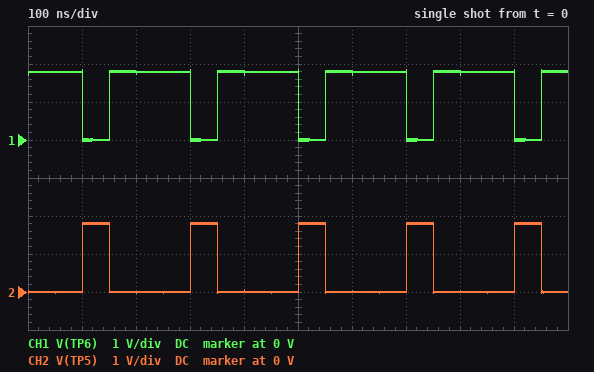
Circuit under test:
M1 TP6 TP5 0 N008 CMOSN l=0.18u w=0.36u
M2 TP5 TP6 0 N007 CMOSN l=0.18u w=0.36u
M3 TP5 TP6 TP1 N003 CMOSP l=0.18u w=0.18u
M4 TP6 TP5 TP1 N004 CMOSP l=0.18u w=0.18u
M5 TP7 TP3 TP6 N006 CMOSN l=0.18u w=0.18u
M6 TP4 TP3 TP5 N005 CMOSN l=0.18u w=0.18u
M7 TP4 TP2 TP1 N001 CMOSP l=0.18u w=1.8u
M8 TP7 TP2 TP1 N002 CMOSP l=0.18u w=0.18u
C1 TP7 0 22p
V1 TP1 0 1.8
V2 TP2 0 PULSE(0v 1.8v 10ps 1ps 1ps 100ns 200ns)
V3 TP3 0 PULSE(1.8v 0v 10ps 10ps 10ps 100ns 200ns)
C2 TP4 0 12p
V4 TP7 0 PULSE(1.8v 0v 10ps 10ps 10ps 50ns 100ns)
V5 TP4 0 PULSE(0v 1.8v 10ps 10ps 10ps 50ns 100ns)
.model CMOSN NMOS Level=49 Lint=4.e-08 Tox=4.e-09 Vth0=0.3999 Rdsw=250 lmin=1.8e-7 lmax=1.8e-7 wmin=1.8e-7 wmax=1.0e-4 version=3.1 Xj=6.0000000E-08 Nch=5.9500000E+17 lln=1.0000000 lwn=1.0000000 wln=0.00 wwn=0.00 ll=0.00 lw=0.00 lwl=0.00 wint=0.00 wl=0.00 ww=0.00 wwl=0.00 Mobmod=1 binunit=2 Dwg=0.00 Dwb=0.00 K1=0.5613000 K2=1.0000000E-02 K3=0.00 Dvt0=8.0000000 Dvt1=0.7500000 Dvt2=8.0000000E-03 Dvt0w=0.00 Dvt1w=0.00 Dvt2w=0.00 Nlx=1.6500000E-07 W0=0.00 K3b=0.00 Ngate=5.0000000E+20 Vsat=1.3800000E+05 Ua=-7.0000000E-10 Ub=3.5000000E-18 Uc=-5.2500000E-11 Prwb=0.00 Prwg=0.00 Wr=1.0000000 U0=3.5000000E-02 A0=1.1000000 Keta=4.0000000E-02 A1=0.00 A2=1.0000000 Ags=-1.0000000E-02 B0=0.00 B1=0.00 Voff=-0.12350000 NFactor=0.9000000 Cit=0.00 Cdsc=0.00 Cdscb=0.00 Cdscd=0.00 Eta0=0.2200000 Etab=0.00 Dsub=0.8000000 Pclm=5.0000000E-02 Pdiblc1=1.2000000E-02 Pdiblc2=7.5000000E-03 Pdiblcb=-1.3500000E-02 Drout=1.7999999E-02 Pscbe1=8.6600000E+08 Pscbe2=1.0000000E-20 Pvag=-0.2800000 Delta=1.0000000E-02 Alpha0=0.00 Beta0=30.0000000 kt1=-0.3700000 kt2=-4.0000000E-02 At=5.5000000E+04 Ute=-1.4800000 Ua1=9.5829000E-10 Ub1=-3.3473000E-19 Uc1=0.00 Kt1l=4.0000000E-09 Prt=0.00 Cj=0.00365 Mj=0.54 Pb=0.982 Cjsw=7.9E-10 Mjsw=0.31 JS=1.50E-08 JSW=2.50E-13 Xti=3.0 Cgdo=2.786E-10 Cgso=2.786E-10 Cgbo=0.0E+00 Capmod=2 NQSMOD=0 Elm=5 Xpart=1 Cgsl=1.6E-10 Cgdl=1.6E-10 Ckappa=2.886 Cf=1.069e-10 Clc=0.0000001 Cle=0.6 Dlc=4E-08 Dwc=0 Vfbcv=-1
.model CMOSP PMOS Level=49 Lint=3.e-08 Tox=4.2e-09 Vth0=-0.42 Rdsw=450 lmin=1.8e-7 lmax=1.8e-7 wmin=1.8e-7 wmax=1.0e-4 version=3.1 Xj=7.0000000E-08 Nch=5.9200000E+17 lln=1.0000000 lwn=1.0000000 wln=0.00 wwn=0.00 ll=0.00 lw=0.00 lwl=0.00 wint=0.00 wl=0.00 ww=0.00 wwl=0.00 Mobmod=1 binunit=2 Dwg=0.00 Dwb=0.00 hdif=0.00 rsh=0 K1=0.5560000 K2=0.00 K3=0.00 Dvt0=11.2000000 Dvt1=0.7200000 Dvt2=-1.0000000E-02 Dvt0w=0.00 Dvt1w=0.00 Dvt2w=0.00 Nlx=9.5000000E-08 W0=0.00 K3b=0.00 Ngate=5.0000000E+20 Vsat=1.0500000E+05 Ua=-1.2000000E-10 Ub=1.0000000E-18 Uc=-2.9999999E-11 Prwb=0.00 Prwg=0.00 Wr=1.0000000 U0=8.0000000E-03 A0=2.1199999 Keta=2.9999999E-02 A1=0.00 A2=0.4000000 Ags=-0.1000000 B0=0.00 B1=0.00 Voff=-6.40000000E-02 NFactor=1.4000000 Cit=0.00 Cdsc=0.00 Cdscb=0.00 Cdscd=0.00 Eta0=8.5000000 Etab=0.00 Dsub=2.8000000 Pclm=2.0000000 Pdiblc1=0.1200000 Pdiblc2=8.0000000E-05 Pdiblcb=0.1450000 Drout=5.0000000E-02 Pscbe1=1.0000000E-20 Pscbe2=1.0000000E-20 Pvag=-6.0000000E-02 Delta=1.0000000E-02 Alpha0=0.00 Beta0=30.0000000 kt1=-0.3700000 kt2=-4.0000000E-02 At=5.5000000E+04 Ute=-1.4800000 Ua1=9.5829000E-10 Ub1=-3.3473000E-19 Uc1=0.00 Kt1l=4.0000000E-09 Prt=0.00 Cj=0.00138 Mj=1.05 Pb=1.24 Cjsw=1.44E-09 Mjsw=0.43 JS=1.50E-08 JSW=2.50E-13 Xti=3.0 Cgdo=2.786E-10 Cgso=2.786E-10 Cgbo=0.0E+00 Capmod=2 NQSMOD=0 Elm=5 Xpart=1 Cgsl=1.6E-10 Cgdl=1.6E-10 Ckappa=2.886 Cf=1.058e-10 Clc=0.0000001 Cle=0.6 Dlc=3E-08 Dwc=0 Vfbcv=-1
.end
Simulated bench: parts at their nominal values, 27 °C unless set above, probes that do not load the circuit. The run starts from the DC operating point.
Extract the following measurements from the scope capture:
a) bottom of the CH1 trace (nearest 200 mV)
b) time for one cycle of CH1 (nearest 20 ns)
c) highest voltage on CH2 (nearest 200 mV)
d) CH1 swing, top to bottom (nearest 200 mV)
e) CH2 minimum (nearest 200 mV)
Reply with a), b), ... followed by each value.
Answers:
a) 0 V
b) 200 ns
c) 1.8 V
d) 1.8 V
e) 0 V
